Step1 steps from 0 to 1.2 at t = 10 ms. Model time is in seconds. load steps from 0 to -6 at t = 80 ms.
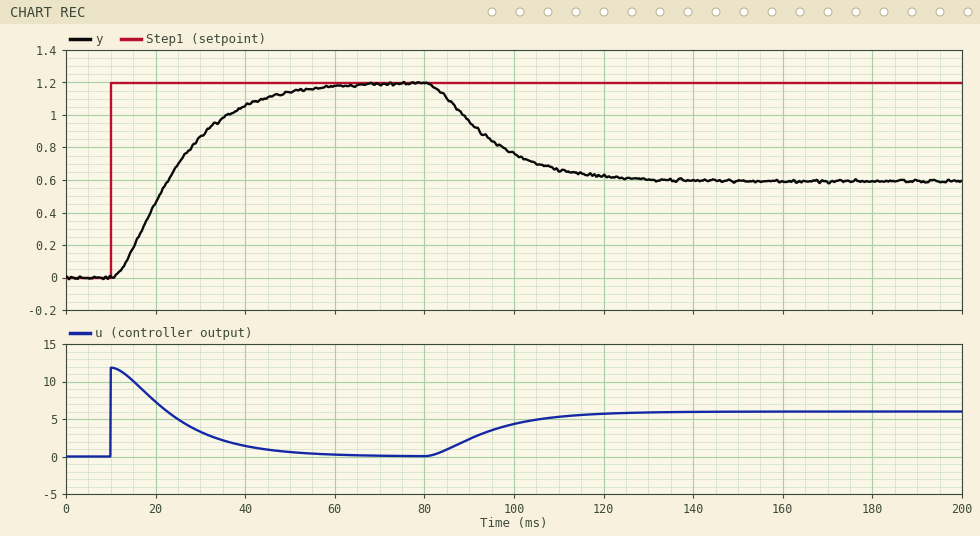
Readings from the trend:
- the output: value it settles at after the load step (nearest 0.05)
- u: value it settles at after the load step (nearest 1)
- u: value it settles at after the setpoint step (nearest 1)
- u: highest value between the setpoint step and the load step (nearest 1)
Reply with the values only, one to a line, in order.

0.60
6
0
12
